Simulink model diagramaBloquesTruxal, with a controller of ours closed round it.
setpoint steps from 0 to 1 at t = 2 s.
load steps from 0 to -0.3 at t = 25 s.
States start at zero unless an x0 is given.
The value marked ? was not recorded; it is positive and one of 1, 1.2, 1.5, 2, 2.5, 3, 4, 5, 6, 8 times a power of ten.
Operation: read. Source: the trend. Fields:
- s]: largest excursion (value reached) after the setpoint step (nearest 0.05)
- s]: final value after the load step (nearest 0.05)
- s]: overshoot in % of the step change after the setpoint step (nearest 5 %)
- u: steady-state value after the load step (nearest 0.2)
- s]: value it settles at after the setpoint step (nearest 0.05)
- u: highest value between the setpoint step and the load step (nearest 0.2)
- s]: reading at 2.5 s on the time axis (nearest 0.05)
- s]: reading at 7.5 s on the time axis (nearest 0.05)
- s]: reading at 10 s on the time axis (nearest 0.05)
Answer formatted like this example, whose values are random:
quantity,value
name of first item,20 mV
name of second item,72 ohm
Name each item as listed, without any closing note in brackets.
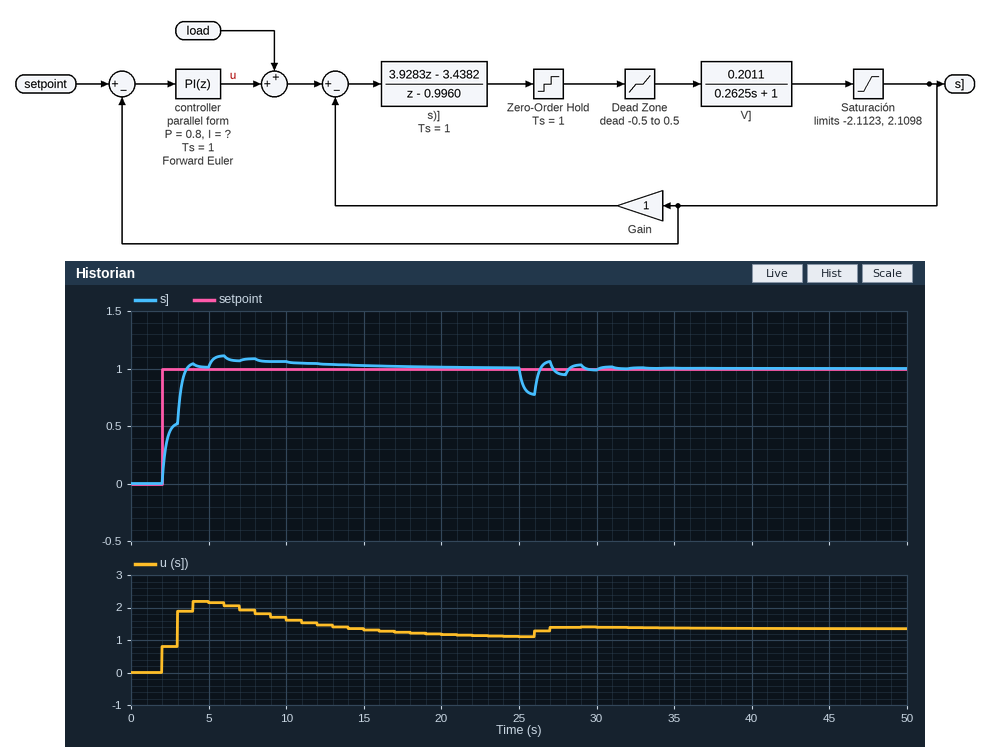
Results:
quantity,value
s]: largest excursion (value reached) after the setpoint step,1.10
s]: final value after the load step,1.00
s]: overshoot in % of the step change after the setpoint step,10 %
u: steady-state value after the load step,1.4
s]: value it settles at after the setpoint step,1.00
u: highest value between the setpoint step and the load step,2.2
s]: reading at 2.5 s on the time axis,0.45
s]: reading at 7.5 s on the time axis,1.10
s]: reading at 10 s on the time axis,1.05
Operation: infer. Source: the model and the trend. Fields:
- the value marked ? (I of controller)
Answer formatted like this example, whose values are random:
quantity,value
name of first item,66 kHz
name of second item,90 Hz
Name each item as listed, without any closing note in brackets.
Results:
quantity,value
the value marked ?,1.5
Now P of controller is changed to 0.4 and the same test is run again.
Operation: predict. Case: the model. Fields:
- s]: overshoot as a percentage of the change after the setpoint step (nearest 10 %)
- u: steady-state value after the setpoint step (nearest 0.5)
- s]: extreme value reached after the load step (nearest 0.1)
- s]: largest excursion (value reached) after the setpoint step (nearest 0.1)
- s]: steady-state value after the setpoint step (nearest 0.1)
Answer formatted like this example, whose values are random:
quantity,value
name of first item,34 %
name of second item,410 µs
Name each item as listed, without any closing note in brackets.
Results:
quantity,value
s]: overshoot as a percentage of the change after the setpoint step,20 %
u: steady-state value after the setpoint step,1.0
s]: extreme value reached after the load step,0.8
s]: largest excursion (value reached) after the setpoint step,1.2
s]: steady-state value after the setpoint step,1.0
